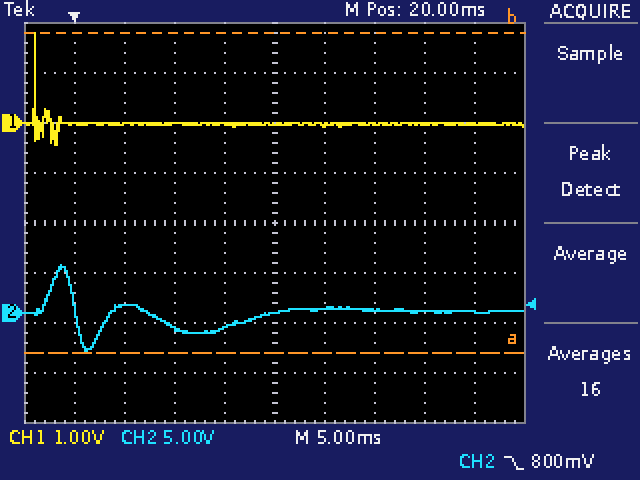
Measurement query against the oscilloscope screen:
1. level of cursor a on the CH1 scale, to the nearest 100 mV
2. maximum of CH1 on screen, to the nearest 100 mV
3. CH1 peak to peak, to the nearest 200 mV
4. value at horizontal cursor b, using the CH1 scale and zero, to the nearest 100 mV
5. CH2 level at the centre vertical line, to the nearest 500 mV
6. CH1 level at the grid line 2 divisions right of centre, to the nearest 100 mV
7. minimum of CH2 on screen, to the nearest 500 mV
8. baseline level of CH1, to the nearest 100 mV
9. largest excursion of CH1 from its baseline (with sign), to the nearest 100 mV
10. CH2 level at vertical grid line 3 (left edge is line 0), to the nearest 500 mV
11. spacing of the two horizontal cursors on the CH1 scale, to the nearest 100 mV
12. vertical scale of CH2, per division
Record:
-4.6 V
1.8 V
2.2 V
1.8 V
0.0 V
0.0 V
-4.0 V
0.0 V
+1.8 V
-1.5 V
6.4 V
5 V
